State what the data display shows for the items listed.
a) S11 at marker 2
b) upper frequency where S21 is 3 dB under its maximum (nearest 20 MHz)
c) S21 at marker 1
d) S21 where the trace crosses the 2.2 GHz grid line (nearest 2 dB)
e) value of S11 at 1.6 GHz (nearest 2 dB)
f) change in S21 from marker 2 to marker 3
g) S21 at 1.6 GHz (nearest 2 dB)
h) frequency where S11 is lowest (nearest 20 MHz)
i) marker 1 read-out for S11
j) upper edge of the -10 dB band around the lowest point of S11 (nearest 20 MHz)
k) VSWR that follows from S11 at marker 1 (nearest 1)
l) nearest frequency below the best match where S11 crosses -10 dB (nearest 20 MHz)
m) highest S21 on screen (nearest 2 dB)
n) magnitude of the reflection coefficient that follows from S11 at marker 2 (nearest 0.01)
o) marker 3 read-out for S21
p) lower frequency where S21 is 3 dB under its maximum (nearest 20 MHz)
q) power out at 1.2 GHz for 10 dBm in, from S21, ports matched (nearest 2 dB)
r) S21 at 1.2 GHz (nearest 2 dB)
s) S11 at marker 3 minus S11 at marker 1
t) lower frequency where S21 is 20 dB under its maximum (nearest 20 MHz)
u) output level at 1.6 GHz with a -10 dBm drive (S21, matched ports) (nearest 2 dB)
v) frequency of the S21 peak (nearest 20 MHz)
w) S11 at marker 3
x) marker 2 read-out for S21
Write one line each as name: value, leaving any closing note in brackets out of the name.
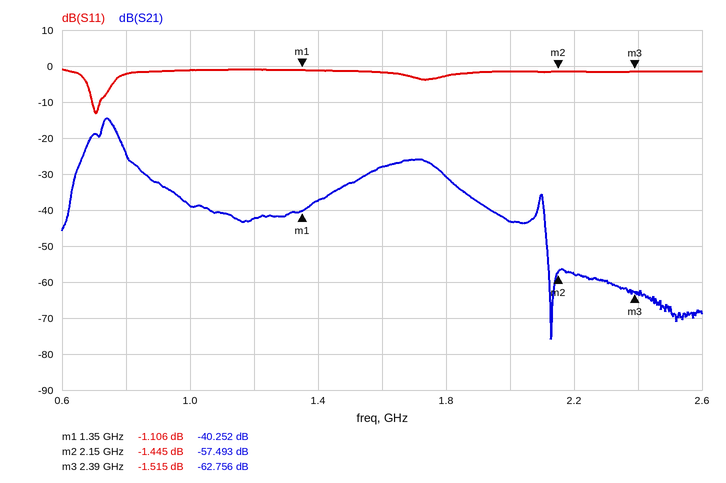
S11 at marker 2: -1.445 dB
upper frequency where S21 is 3 dB under its maximum: 760 MHz
S21 at marker 1: -40.252 dB
S21 where the trace crosses the 2.2 GHz grid line: -58 dB
value of S11 at 1.6 GHz: -2 dB
change in S21 from marker 2 to marker 3: -5.263 dB
S21 at 1.6 GHz: -28 dB
frequency where S11 is lowest: 700 MHz
marker 1 read-out for S11: -1.106 dB
upper edge of the -10 dB band around the lowest point of S11: 720 MHz
VSWR that follows from S11 at marker 1: 16
nearest frequency below the best match where S11 crosses -10 dB: 700 MHz
highest S21 on screen: -14 dB
magnitude of the reflection coefficient that follows from S11 at marker 2: 0.85
marker 3 read-out for S21: -62.756 dB
lower frequency where S21 is 3 dB under its maximum: 720 MHz
power out at 1.2 GHz for 10 dBm in, from S21, ports matched: -32 dBm
S21 at 1.2 GHz: -42 dB
S11 at marker 3 minus S11 at marker 1: -0.409 dB
lower frequency where S21 is 20 dB under its maximum: 640 MHz
output level at 1.6 GHz with a -10 dBm drive (S21, matched ports): -38 dBm
frequency of the S21 peak: 740 MHz
S11 at marker 3: -1.515 dB
marker 2 read-out for S21: -57.493 dB
